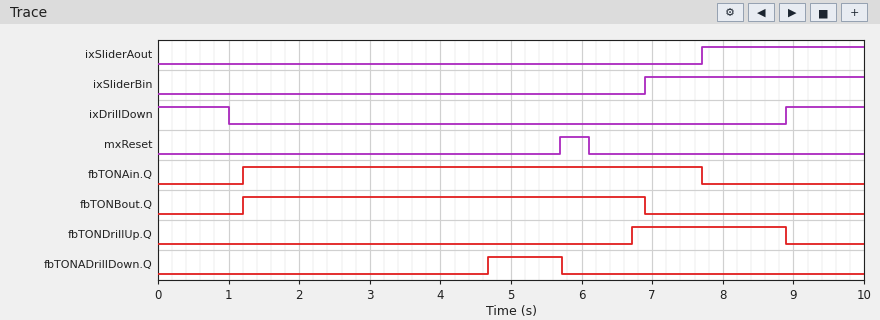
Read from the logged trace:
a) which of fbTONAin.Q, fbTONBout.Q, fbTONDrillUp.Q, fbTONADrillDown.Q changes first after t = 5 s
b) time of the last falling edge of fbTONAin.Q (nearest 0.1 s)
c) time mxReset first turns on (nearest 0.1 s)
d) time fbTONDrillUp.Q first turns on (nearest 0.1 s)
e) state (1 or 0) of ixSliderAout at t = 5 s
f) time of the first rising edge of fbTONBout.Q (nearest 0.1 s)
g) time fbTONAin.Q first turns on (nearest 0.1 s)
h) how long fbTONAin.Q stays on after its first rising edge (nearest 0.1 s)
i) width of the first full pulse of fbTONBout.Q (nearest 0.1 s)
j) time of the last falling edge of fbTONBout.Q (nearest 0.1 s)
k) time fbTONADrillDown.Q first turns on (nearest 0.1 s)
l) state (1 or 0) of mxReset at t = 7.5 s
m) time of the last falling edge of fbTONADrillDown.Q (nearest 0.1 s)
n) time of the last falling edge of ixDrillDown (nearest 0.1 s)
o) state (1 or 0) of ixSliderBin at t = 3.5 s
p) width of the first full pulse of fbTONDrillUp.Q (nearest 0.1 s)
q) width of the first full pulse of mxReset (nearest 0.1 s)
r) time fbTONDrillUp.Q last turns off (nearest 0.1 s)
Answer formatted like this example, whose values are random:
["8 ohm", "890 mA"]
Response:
["fbTONADrillDown.Q", "7.7 s", "5.7 s", "6.7 s", "0", "1.2 s", "1.2 s", "6.5 s", "5.7 s", "6.9 s", "4.7 s", "0", "5.7 s", "1.0 s", "0", "2.2 s", "0.4 s", "8.9 s"]
